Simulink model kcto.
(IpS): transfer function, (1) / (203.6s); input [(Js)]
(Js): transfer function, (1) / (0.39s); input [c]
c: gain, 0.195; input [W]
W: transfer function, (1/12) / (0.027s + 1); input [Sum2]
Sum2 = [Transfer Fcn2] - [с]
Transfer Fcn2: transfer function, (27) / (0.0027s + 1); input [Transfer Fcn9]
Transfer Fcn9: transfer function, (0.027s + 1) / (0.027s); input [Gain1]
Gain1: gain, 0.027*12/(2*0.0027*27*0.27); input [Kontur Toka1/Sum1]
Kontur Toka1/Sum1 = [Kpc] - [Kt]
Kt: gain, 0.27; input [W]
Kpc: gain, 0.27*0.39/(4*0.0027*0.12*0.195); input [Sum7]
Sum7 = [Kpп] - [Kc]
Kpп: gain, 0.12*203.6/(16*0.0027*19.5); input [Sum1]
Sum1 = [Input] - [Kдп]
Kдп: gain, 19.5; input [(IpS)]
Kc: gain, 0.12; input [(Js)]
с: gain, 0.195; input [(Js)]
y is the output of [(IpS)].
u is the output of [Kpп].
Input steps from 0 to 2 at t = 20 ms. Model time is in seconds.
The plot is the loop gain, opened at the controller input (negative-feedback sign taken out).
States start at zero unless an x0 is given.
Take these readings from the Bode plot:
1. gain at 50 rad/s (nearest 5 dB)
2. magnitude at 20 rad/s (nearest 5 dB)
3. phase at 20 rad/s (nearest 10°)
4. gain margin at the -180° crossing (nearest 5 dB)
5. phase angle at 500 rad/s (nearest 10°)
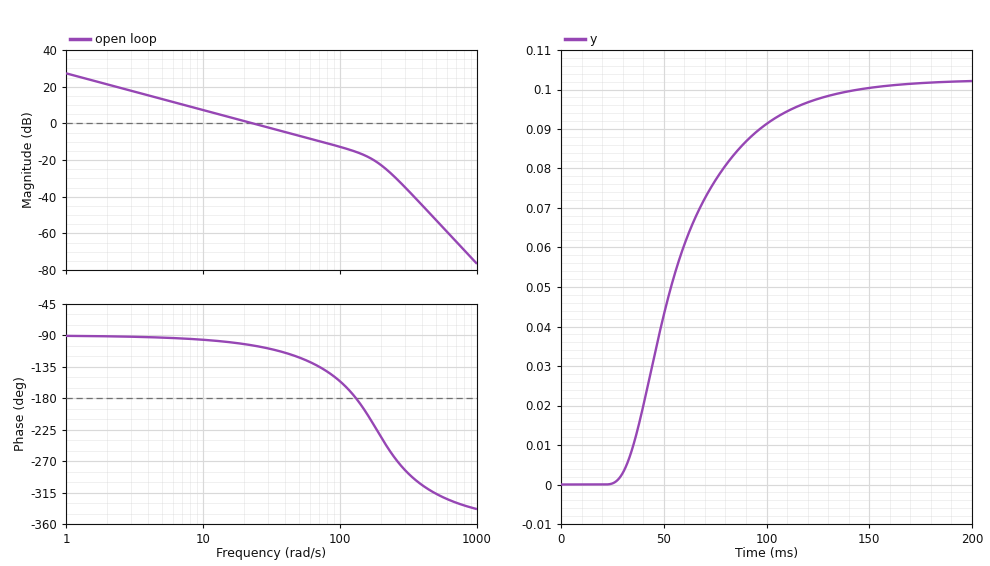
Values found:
-5 dB
0 dB
-100°
15 dB
-320°
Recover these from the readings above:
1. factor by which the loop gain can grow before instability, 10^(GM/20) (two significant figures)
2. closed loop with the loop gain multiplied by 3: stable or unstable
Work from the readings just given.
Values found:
5.6
stable
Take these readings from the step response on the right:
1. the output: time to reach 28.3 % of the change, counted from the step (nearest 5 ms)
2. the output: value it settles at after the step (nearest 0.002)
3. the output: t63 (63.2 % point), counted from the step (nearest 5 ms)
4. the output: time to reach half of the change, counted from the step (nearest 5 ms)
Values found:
25 ms
0.102
45 ms
35 ms
